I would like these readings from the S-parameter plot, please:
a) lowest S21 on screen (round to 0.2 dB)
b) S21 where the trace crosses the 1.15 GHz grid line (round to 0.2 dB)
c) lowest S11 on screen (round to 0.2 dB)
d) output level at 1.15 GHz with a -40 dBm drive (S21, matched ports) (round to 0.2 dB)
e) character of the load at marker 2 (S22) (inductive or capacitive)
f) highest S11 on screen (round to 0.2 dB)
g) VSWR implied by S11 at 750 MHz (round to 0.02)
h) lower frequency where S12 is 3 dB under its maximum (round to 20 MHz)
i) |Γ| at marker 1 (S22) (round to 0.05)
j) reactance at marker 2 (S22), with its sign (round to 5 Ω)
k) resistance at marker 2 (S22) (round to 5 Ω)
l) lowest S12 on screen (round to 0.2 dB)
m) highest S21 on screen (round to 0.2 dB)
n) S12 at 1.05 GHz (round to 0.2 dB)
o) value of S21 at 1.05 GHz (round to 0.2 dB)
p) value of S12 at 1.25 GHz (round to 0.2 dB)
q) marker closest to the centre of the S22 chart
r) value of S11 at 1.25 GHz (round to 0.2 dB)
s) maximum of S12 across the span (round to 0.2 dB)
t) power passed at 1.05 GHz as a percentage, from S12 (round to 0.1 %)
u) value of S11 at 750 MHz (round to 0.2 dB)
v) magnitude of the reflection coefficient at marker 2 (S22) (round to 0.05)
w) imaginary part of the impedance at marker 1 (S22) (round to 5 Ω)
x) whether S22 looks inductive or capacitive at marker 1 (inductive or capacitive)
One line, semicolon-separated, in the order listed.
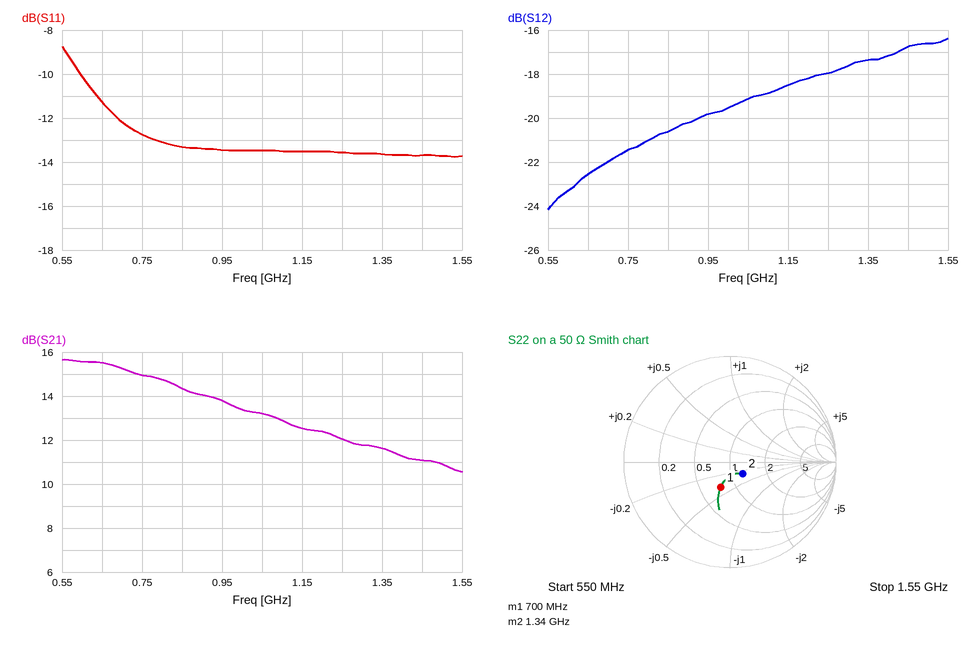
10.6 dB; 12.6 dB; -13.8 dB; -27.4 dBm; capacitive; -8.8 dB; 1.60; 1.02 GHz; 0.25; -15 Ω; 60 Ω; -24.2 dB; 15.6 dB; -19.2 dB; 13.2 dB; -18.0 dB; marker 2; -13.6 dB; -16.4 dB; 1.2 %; -12.8 dB; 0.15; -20 Ω; capacitive
